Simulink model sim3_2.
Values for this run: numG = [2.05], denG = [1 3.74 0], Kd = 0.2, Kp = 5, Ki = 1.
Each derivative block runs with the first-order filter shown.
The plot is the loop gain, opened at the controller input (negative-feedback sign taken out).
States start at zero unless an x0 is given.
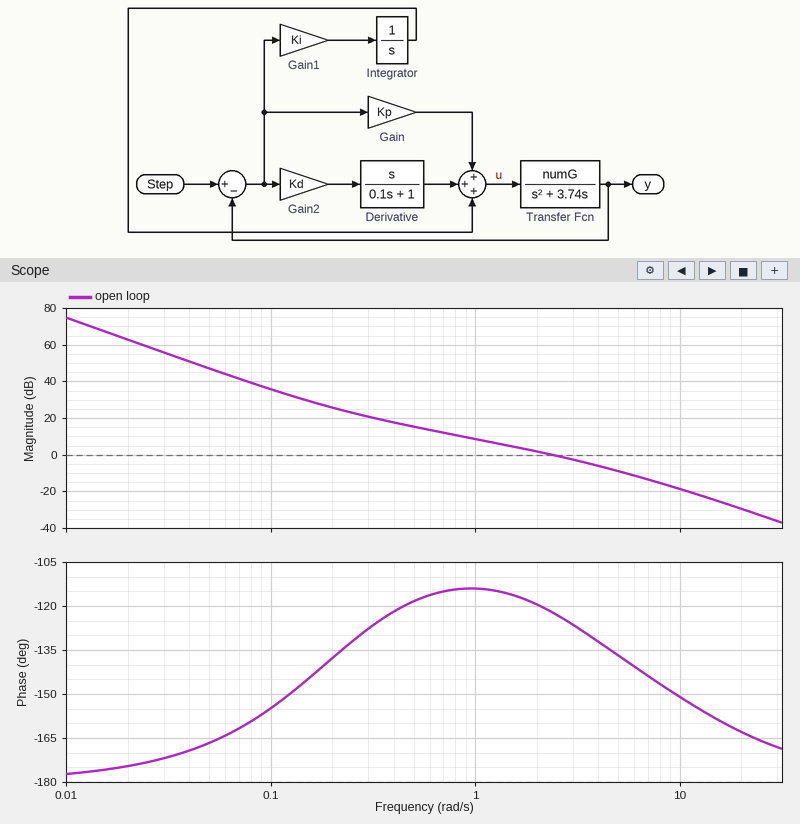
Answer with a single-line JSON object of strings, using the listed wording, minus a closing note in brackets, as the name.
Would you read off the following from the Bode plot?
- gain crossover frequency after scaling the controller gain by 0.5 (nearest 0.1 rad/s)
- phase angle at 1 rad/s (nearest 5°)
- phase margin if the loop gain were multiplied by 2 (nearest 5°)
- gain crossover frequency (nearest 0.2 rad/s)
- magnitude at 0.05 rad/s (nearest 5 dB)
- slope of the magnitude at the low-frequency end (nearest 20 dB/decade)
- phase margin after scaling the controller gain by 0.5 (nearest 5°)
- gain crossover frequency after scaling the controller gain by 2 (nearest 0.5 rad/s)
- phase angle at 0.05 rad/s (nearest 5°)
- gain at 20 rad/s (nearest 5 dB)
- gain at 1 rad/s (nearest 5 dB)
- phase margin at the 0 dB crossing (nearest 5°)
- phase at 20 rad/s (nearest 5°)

{"gain crossover frequency after scaling the controller gain by 0.5": "1.3 rad/s", "phase angle at 1 rad/s": "-115°", "phase margin if the loop gain were multiplied by 2": "50°", "gain crossover frequency": "2.4 rad/s", "magnitude at 0.05 rad/s": "45 dB", "slope of the magnitude at the low-frequency end": "-40 dB/decade", "phase margin after scaling the controller gain by 0.5": "65°", "gain crossover frequency after scaling the controller gain by 2": "4.0 rad/s", "phase angle at 0.05 rad/s": "-165°", "gain at 20 rad/s": "-30 dB", "gain at 1 rad/s": "10 dB", "phase margin at the 0 dB crossing": "60°", "phase at 20 rad/s": "-165°"}
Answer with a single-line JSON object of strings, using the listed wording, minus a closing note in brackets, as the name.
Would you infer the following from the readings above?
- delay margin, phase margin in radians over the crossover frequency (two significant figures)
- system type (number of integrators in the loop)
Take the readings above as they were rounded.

{"delay margin, phase margin in radians over the crossover frequency": "0.44 s", "system type": "2"}
